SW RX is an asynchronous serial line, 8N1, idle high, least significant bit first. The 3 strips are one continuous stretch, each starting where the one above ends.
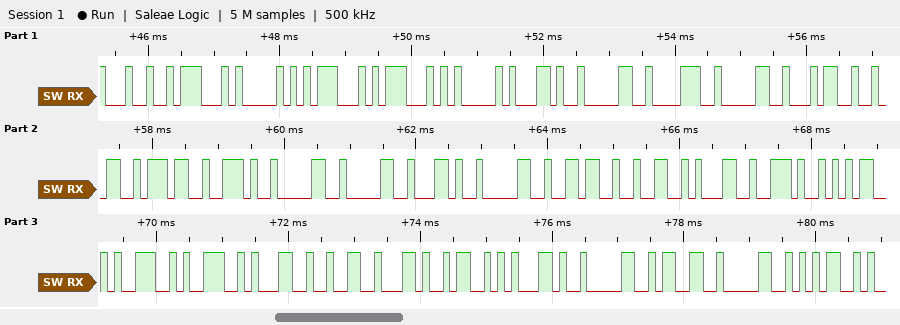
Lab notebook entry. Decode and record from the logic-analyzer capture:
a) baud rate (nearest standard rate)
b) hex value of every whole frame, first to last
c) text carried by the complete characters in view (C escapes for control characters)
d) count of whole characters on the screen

9600 baud
24 47 50 47 47 41 2C 30 38 30 34 32 37 2E 30 30 2C 30 36 32 31 2E 35 39 39 31 32 2C 53 2C 30 33 30 35
"$GPGGA,080427.00,0621.59912,S,0305"
34
